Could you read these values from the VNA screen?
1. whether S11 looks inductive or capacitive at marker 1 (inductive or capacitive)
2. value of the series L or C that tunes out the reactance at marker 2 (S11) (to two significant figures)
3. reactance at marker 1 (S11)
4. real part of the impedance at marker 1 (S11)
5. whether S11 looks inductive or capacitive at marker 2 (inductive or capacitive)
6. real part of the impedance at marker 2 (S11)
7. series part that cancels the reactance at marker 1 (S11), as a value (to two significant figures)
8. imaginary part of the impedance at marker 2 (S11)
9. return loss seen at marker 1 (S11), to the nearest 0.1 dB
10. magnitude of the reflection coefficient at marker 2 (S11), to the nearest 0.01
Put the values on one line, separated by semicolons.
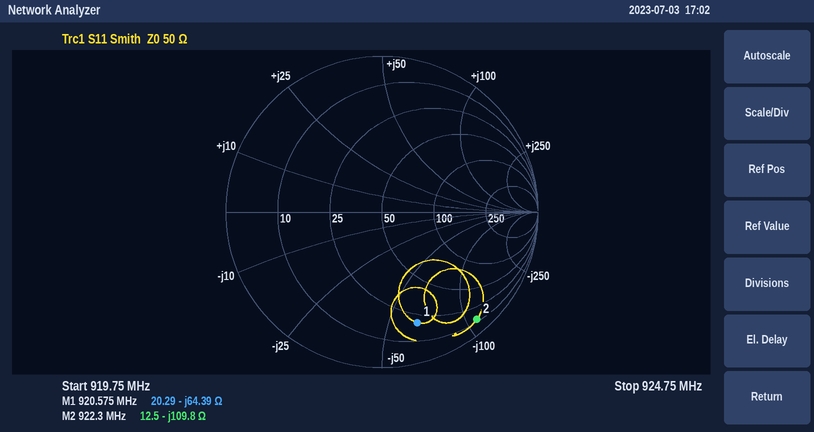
capacitive; 19 nH; -64.39 Ω; 20.29 Ω; capacitive; 12.5 Ω; 11 nH; -109.8 Ω; 2.6 dB; 0.92
